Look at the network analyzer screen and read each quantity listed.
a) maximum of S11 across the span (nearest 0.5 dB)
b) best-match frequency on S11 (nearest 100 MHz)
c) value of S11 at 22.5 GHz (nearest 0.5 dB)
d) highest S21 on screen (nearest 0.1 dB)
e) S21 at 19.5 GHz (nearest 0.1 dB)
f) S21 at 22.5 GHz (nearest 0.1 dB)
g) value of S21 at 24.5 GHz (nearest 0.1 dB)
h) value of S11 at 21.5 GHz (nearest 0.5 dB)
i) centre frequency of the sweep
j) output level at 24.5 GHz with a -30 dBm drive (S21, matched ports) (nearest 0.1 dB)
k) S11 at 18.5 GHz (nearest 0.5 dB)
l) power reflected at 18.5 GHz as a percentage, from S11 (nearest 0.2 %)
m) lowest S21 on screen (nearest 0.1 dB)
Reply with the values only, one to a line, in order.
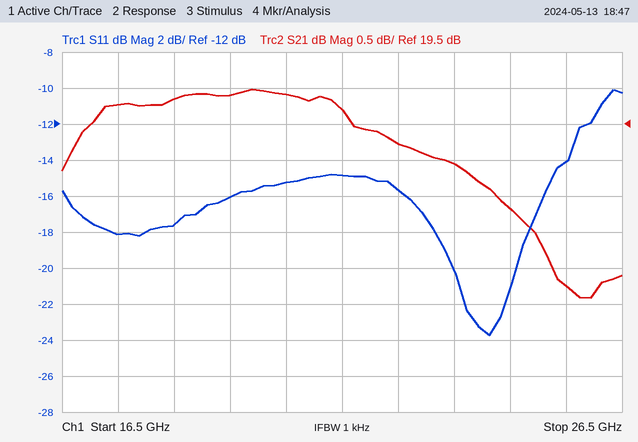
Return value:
-10.0 dB
24.1 GHz
-15.5 dB
20.0 dB
19.9 dB
19.2 dB
18.3 dB
-15.0 dB
21.5 GHz
-11.7 dBm
-17.5 dB
1.8 %
17.1 dB
